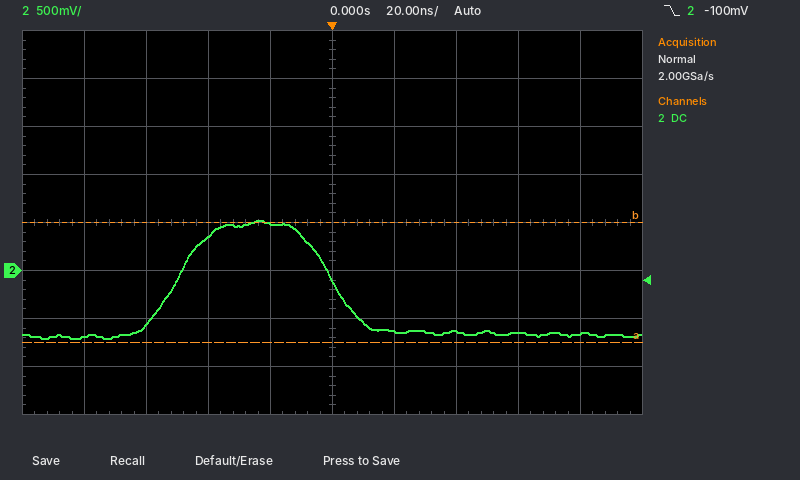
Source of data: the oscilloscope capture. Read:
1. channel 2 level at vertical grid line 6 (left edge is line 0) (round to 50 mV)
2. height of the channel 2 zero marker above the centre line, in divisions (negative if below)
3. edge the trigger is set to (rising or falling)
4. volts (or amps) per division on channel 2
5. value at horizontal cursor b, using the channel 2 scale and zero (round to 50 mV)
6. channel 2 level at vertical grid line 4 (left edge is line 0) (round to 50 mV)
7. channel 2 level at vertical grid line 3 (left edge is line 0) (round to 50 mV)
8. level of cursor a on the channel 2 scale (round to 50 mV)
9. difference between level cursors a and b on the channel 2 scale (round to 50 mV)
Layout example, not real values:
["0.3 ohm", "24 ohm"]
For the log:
["-650 mV", "-1.0 div", "falling", "500 mV", "500 mV", "500 mV", "350 mV", "-750 mV", "1.25 V"]
